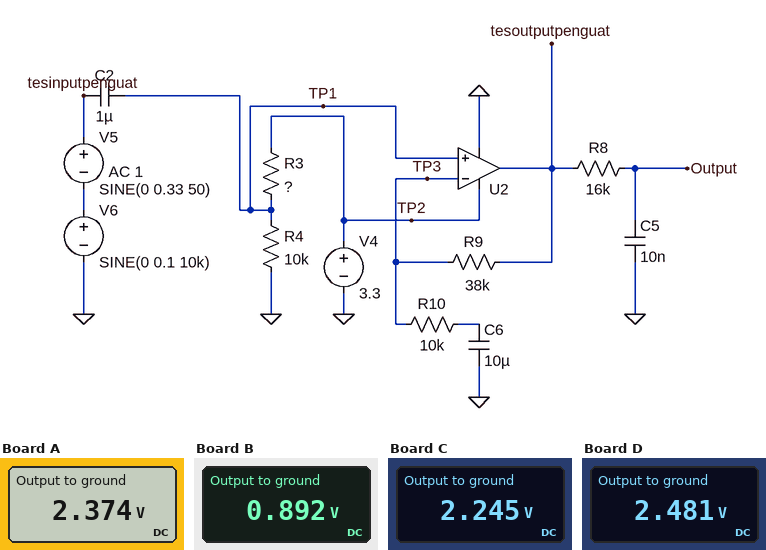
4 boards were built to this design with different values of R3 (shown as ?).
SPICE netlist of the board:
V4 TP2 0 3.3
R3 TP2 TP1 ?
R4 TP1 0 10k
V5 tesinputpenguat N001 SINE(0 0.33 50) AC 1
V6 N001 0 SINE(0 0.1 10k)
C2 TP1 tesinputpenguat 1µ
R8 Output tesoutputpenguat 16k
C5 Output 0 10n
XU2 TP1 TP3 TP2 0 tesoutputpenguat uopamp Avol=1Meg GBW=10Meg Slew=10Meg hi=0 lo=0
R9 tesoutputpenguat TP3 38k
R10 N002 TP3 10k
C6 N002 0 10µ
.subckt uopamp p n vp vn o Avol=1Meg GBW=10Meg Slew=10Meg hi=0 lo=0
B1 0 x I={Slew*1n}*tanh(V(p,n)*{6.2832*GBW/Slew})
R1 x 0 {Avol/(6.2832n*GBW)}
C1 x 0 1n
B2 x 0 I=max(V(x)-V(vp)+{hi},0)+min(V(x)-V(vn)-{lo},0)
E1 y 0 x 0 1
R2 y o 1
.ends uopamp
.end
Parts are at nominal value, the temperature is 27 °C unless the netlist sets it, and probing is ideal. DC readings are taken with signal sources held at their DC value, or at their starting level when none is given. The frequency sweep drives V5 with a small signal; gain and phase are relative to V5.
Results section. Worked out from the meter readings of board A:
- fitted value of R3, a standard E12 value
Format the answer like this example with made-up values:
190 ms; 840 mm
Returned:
3.9 kΩ
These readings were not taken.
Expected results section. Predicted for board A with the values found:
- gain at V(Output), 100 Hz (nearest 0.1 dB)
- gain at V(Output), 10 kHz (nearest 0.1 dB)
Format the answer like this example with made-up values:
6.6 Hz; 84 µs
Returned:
12.4 dB; -6.5 dB
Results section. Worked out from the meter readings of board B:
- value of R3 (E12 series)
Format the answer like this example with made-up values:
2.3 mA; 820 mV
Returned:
27 kΩ
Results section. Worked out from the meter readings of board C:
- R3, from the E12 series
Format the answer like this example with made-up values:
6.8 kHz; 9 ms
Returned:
4.7 kΩ
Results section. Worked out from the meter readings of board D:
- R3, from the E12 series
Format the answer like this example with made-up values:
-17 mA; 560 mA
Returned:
3.3 kΩ
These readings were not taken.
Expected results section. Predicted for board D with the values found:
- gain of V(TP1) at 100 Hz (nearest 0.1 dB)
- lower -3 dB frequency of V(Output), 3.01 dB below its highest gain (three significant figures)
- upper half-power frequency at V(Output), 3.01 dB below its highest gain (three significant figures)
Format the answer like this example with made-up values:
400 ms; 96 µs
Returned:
-1.5 dB; 57.2 Hz; 1.12 kHz
